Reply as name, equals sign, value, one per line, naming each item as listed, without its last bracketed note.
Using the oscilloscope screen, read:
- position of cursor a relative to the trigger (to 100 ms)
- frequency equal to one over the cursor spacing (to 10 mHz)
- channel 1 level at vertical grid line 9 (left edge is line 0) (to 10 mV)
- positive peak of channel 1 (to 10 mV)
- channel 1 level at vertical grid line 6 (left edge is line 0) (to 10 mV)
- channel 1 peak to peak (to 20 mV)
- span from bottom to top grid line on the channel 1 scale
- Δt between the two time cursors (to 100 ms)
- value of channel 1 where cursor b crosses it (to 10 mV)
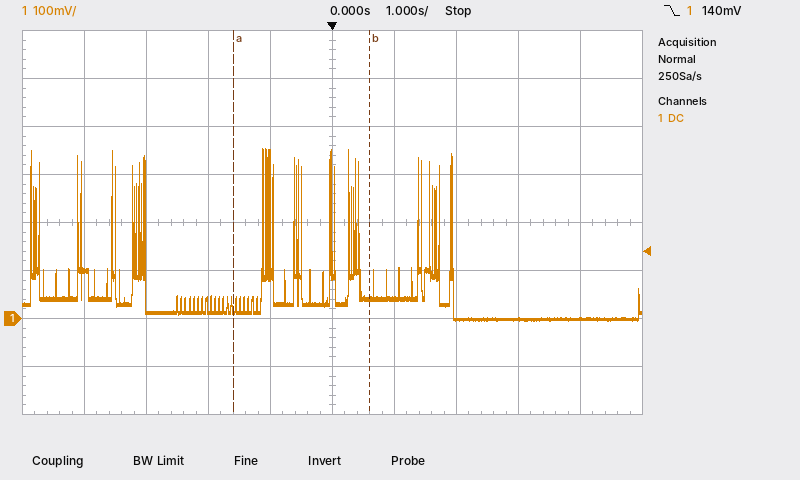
position of cursor a relative to the trigger = -1.6 s
frequency equal to one over the cursor spacing = 450 mHz
channel 1 level at vertical grid line 9 (left edge is line 0) = 0 mV
positive peak of channel 1 = 350 mV
channel 1 level at vertical grid line 6 (left edge is line 0) = 40 mV
channel 1 peak to peak = 360 mV
span from bottom to top grid line on the channel 1 scale = 800 mV
Δt between the two time cursors = 2.2 s
value of channel 1 where cursor b crosses it = 40 mV
